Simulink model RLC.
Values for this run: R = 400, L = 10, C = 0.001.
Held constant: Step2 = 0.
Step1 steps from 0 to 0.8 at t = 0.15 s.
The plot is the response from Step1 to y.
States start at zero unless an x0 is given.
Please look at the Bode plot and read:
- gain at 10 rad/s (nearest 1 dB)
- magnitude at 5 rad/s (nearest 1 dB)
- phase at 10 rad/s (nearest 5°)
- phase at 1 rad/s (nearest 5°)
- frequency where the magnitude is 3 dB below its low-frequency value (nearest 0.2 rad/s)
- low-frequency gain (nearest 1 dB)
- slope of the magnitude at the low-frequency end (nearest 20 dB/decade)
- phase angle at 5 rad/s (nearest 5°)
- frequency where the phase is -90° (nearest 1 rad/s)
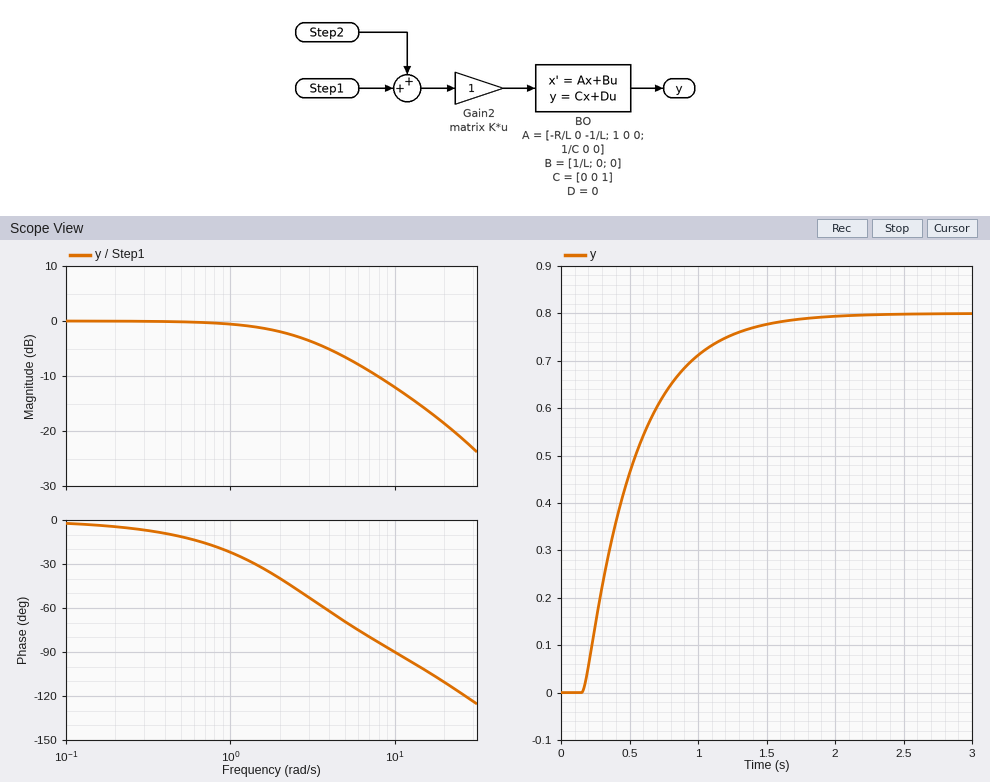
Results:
-12 dB
-7 dB
-90°
-20°
2.6 rad/s
0 dB
0 dB/decade
-70°
10 rad/s
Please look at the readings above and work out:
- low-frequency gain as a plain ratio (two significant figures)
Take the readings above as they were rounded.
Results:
1.0
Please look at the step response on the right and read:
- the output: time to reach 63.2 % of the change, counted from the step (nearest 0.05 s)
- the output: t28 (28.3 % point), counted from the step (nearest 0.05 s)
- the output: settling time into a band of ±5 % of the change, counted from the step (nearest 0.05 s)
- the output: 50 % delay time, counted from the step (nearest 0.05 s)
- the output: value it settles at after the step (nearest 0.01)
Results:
0.40 s
0.15 s
1.15 s
0.30 s
0.80
